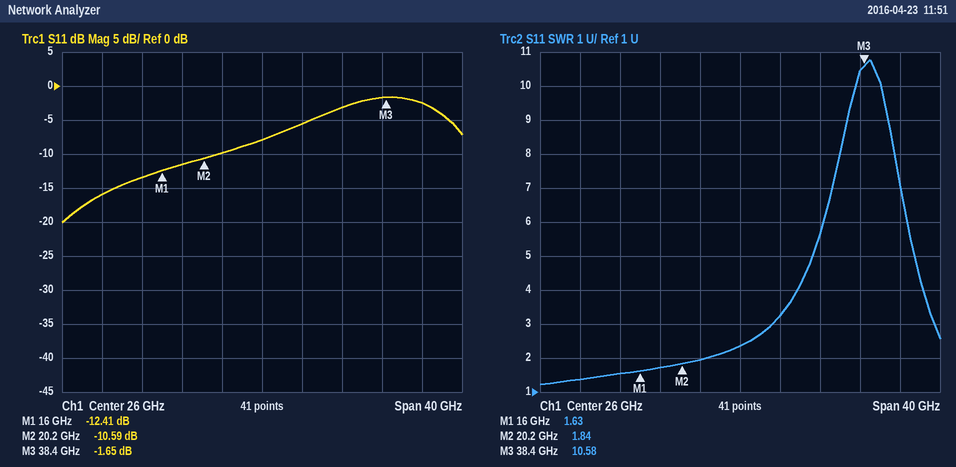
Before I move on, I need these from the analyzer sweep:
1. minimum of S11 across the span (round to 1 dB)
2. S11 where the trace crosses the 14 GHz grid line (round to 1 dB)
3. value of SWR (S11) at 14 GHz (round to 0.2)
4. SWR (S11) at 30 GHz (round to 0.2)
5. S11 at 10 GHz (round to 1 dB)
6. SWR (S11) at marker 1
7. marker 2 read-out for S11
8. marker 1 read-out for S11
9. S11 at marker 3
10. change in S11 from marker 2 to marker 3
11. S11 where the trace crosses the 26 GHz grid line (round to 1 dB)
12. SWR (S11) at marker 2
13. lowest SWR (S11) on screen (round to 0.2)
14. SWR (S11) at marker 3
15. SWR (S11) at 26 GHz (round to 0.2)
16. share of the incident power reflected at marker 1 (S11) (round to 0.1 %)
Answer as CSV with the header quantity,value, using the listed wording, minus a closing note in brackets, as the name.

quantity,value
minimum of S11 across the span,-20 dB
S11 where the trace crosses the 14 GHz grid line,-13 dB
value of SWR (S11) at 14 GHz,1.6
SWR (S11) at 30 GHz,3.2
S11 at 10 GHz,-16 dB
SWR (S11) at marker 1,1.63
marker 2 read-out for S11,-10.59 dB
marker 1 read-out for S11,-12.41 dB
S11 at marker 3,-1.65 dB
change in S11 from marker 2 to marker 3,8.94 dB
S11 where the trace crosses the 26 GHz grid line,-8 dB
SWR (S11) at marker 2,1.84
lowest SWR (S11) on screen,1.2
SWR (S11) at marker 3,10.58
SWR (S11) at 26 GHz,2.4
share of the incident power reflected at marker 1 (S11),5.7 %
